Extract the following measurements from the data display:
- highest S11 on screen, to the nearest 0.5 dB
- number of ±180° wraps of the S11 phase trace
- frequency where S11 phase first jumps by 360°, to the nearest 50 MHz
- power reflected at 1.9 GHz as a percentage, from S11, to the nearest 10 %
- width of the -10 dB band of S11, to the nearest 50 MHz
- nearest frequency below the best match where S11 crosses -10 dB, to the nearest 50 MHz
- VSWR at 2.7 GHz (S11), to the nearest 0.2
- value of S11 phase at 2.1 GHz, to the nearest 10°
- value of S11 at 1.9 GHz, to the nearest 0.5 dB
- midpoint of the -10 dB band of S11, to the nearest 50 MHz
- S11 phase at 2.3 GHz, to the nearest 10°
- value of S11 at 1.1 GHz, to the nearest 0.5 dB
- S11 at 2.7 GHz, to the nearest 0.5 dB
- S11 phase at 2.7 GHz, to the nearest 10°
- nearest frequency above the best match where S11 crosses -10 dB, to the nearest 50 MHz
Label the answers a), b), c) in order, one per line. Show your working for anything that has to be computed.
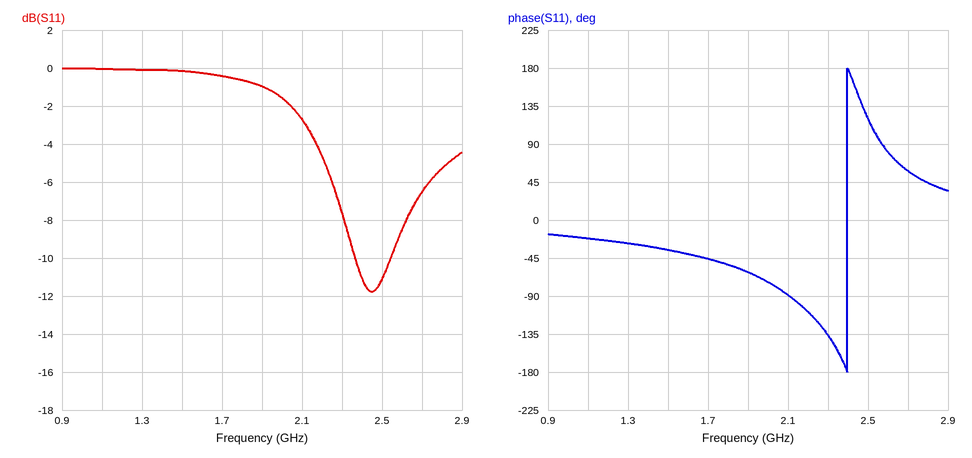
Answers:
a) 0.0 dB
b) 1
c) 2.40 GHz
d) 10^(-1/10) ≈ 79.4 %, so 80 % to the nearest 10 %
e) 2.55 GHz − 2.35 GHz = 200 MHz
f) 2.35 GHz
g) |Γ| = 10^(-6.5/20) = 0.4732; VSWR = (1 + 0.4732)/(1 − 0.4732) ≈ 2.8
h) -90°
i) -1.0 dB
j) 2.45 GHz
k) -140°
l) 0.0 dB
m) -6.5 dB
n) 60°
o) 2.55 GHz
